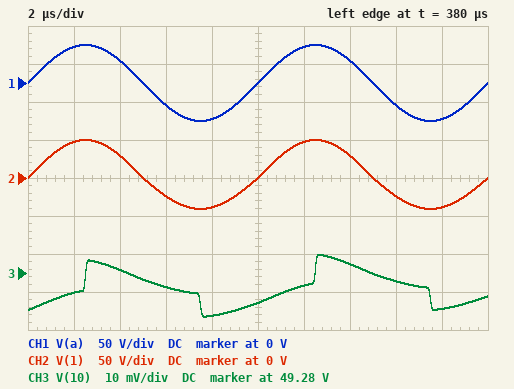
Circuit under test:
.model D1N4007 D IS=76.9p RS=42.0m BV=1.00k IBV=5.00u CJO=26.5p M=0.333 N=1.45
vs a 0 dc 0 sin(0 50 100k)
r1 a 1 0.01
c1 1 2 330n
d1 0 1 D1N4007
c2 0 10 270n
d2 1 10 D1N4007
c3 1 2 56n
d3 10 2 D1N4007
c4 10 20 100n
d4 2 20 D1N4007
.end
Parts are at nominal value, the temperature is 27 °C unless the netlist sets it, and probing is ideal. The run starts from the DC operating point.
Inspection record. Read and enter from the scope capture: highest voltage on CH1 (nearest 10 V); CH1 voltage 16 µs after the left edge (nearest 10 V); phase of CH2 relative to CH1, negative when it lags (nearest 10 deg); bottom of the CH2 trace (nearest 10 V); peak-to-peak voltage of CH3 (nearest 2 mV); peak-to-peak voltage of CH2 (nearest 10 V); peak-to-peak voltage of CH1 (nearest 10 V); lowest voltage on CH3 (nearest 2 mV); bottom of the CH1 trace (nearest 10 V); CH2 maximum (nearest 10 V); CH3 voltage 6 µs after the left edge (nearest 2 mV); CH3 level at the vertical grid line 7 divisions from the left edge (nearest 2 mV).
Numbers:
50 V
-30 V
0 deg
-40 V
16 mV
90 V
100 V
49.268 V
-50 V
50 V
49.276 V
49.282 V
